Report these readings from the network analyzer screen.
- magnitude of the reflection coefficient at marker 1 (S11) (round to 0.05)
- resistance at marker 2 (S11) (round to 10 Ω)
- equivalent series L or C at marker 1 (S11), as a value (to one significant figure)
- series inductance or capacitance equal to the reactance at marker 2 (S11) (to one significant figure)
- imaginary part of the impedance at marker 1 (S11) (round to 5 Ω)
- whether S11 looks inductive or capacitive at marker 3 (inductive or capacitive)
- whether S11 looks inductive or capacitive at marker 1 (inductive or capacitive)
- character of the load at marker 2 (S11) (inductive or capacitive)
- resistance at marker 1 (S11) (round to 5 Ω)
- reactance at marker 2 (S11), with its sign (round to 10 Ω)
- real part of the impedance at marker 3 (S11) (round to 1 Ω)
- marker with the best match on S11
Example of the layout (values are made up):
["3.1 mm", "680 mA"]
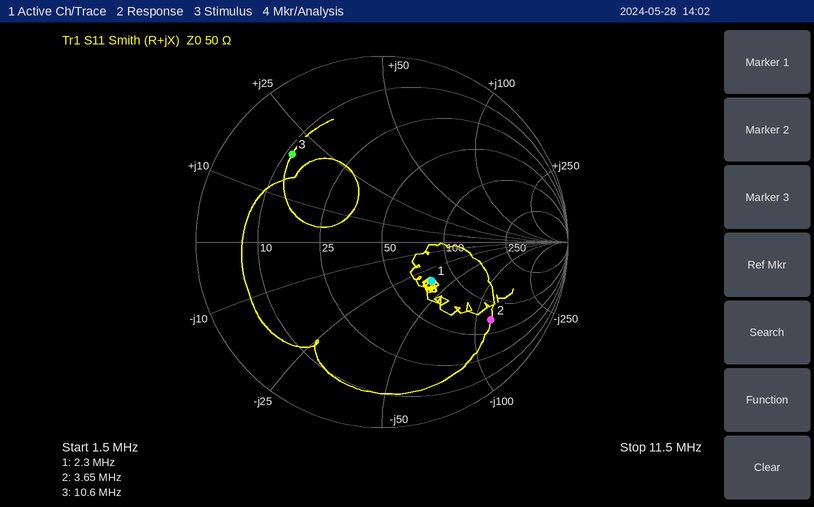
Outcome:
["0.35", "70 Ω", "2 nF", "400 pF", "-35 Ω", "inductive", "capacitive", "capacitive", "75 Ω", "-120 Ω", "11 Ω", "marker 1"]
